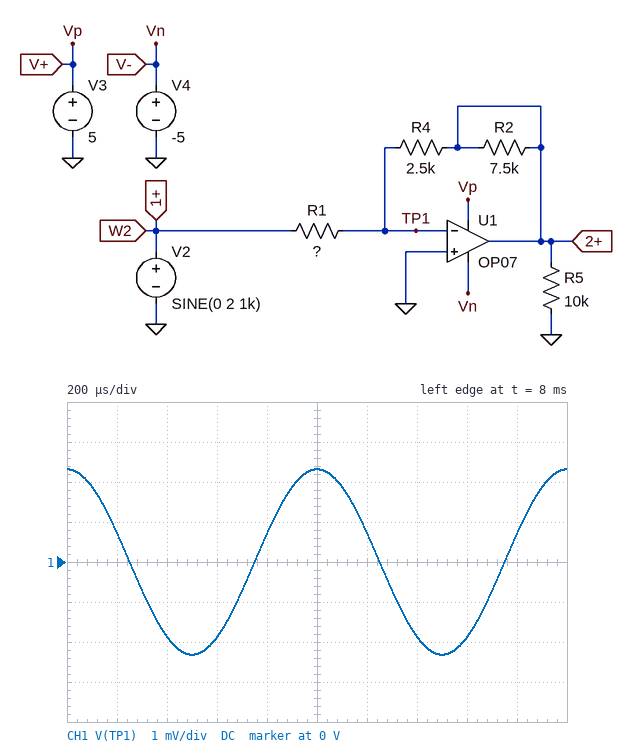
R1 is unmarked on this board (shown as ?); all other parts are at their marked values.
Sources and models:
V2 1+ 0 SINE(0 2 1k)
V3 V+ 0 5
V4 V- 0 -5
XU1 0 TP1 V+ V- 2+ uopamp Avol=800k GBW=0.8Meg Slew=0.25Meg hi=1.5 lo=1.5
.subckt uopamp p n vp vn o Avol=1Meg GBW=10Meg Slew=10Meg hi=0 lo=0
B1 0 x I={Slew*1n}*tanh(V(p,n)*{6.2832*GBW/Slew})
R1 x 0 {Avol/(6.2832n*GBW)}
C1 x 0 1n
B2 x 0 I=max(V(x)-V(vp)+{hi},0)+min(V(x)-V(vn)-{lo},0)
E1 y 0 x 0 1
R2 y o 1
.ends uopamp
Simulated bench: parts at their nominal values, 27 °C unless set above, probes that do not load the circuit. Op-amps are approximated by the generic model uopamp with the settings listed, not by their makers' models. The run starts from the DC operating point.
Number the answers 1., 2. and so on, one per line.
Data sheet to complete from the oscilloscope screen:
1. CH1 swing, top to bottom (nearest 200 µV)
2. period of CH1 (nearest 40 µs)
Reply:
1. 4.6 mV
2. 1.00 ms
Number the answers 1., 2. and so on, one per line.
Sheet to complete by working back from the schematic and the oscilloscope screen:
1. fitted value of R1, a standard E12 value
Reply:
1. 2.7 kΩ
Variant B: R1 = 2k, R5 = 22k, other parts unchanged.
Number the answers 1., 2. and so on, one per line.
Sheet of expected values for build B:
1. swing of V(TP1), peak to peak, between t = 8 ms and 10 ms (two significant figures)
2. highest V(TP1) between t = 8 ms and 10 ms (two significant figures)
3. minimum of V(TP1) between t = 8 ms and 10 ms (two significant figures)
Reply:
1. 6.3 mV
2. 3.1 mV
3. -3.1 mV
